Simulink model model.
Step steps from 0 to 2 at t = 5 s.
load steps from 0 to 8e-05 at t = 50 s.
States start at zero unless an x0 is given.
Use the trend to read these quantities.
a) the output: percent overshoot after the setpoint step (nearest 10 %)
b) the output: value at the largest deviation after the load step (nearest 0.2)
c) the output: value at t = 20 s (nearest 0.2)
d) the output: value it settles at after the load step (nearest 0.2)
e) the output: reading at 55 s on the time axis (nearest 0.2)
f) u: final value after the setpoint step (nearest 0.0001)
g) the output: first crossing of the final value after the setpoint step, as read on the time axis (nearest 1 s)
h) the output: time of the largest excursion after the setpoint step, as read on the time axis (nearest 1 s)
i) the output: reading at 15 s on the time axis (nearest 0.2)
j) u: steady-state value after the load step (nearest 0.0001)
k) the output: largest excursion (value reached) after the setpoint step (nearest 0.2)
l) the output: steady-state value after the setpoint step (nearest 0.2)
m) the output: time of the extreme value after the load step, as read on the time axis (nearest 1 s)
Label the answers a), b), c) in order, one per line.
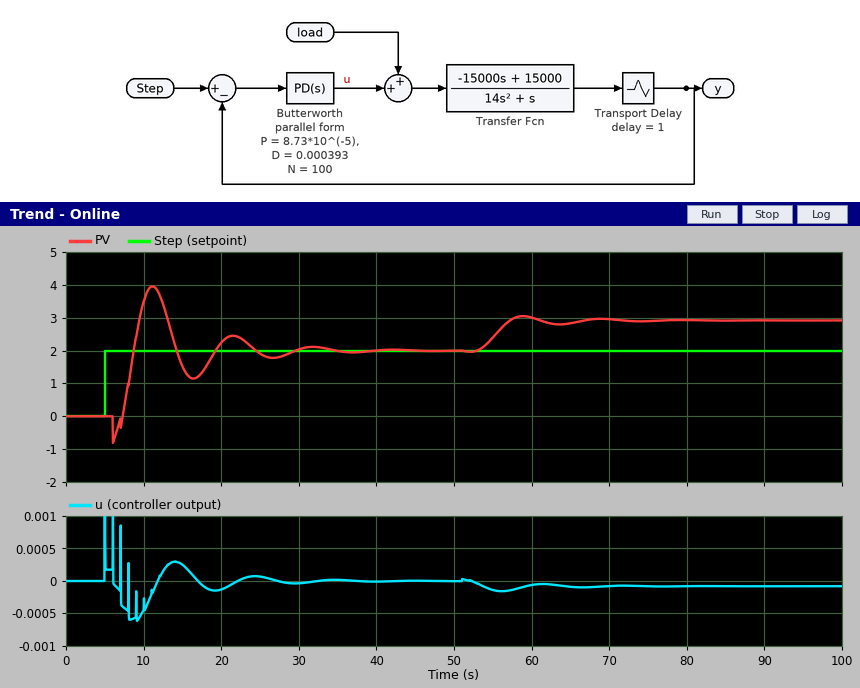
a) 100 %
b) 3.0
c) 2.2
d) 3.0
e) 2.4
f) 0.0000
g) 9 s
h) 11 s
i) 1.6
j) -0.0001
k) 4.0
l) 2.0
m) 59 s
